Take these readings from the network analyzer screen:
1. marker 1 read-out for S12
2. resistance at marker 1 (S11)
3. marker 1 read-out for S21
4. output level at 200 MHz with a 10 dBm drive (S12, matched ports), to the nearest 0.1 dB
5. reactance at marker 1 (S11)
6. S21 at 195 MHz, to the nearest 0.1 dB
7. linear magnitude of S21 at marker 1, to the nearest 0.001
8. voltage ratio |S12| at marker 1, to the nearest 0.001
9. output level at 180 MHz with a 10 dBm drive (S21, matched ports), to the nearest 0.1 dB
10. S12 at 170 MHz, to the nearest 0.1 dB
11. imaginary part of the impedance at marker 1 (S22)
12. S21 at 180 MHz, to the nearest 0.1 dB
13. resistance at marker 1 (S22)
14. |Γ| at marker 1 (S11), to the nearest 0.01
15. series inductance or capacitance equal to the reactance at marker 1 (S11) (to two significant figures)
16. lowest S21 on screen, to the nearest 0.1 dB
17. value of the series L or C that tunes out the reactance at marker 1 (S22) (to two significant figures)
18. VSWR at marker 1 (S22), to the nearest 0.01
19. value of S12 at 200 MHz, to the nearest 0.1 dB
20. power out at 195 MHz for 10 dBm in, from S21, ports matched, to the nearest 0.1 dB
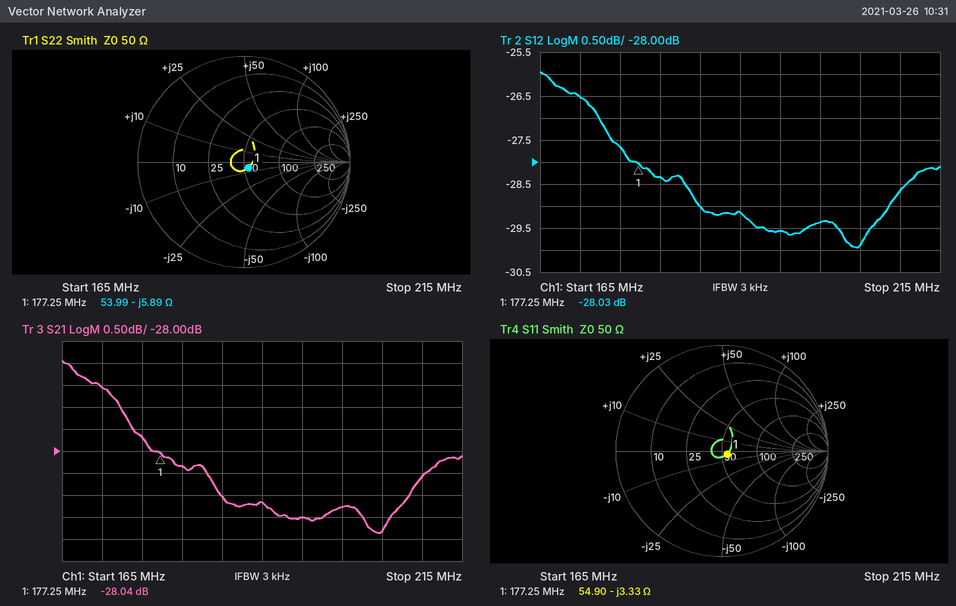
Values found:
-28.03 dB
54.90 Ω
-28.04 dB
-19.4 dBm
-3.33 Ω
-29.5 dB
0.040
0.040
-18.3 dBm
-26.5 dB
-5.89 Ω
-28.3 dB
53.99 Ω
0.06
270 pF
-29.9 dB
5.3 nH
1.15
-29.4 dB
-19.5 dBm
